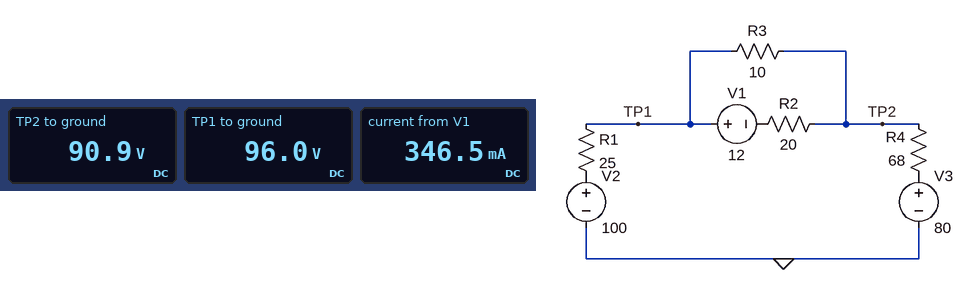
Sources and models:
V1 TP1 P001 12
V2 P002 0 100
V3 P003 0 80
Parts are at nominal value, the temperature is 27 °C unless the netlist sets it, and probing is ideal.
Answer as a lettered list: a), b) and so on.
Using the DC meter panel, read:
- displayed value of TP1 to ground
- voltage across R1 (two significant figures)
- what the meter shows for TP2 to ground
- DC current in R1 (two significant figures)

a) 96.0 V
b) 4.0 V
c) 90.9 V
d) 160 mA
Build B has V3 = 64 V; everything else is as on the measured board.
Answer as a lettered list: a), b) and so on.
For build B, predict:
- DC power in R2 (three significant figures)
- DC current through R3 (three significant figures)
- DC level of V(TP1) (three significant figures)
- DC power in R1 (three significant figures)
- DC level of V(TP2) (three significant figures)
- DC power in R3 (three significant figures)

a) 1.72 W
b) 614 mA
c) 92.0 V
d) 2.58 W
e) 85.8 V
f) 3.77 W
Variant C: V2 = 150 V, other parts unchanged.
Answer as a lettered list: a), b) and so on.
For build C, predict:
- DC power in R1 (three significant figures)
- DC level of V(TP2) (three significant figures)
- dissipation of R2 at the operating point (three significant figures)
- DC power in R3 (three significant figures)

a) 11.0 W
b) 125 V
c) 643 mW
d) 7.08 W
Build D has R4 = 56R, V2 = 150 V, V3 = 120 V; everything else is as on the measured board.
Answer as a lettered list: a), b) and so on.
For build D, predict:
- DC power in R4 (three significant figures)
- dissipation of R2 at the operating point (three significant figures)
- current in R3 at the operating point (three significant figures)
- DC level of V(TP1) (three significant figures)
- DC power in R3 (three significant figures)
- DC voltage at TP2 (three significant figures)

a) 4.93 W
b) 1.81 W
c) 598 mA
d) 143 V
e) 3.57 W
f) 137 V
